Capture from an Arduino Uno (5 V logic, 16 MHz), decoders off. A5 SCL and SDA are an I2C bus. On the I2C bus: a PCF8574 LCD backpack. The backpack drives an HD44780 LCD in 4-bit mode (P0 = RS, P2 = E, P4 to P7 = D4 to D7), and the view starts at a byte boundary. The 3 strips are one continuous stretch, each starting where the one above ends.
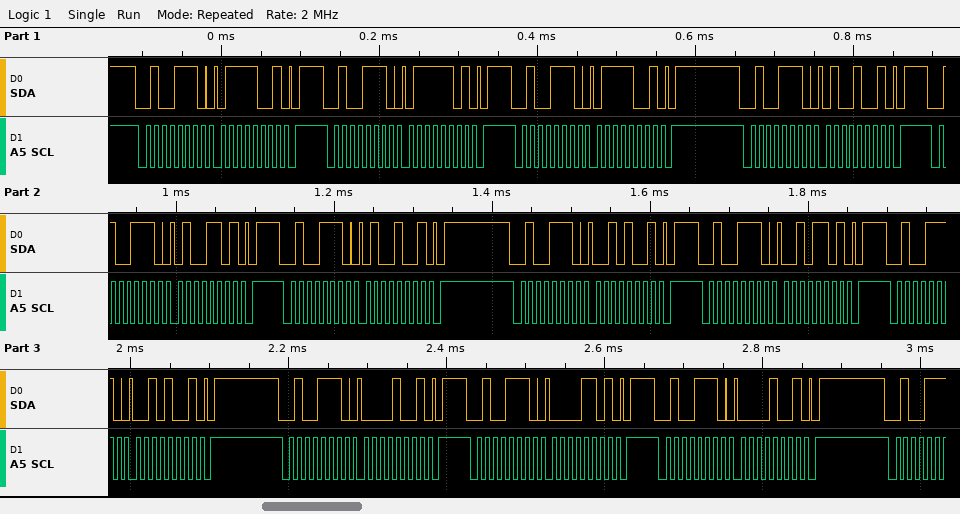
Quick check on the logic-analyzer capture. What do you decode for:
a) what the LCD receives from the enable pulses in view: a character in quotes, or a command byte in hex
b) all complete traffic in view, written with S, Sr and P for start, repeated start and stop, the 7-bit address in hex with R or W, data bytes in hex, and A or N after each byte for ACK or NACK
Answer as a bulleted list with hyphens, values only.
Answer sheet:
- 't' ' '
- S 27W A 79 A P S 27W A 7D A P S 27W A 79 A P S 27W A 49 A P S 27W A 4D A P S 27W A 49 A P S 27W A 29 A P S 27W A 2D A P S 27W A 29 A P S 27W A 09 A P S 27W A 0D A P S 27W A 09 A P
